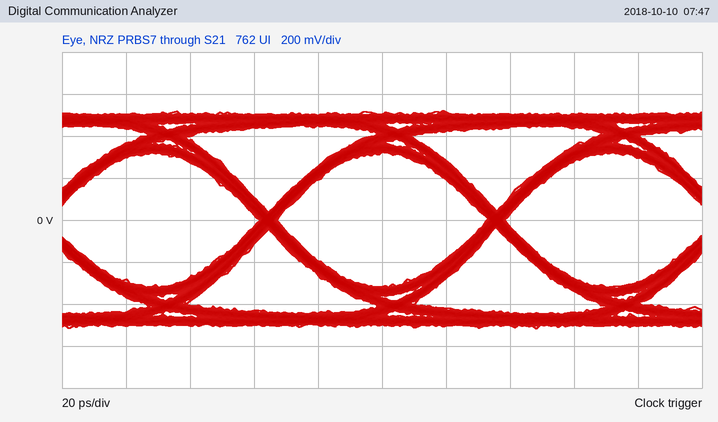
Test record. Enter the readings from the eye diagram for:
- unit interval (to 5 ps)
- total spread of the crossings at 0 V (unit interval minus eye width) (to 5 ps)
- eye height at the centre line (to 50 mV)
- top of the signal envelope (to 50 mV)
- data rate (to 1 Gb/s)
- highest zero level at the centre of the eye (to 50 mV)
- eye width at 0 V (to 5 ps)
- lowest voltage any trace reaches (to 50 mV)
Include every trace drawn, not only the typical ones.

70 ps
5 ps
650 mV
500 mV
14 Gb/s
-300 mV
65 ps
-500 mV
